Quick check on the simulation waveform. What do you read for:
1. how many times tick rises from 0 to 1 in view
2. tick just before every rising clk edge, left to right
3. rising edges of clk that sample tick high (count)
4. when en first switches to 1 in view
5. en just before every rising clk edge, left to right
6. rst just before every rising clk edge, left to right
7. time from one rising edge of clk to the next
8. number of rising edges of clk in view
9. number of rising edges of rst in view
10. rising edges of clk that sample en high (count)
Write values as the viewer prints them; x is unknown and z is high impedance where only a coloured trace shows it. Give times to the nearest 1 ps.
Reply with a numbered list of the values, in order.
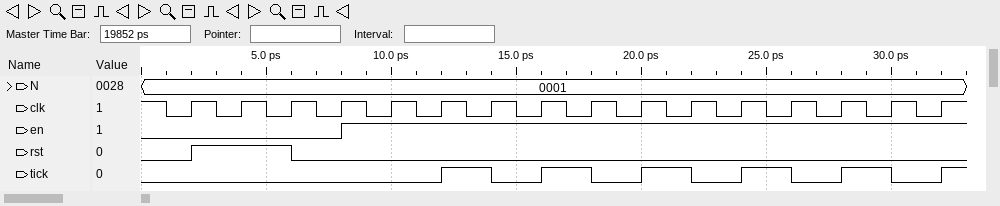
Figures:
1. 6
2. 0 0 0 0 0 0 1 0 1 0 1 0 1 0 1 0
3. 5
4. 8 ps
5. 0 0 0 0 1 1 1 1 1 1 1 1 1 1 1 1
6. 0 1 1 0 0 0 0 0 0 0 0 0 0 0 0 0
7. 2 ps
8. 16
9. 1
10. 12
